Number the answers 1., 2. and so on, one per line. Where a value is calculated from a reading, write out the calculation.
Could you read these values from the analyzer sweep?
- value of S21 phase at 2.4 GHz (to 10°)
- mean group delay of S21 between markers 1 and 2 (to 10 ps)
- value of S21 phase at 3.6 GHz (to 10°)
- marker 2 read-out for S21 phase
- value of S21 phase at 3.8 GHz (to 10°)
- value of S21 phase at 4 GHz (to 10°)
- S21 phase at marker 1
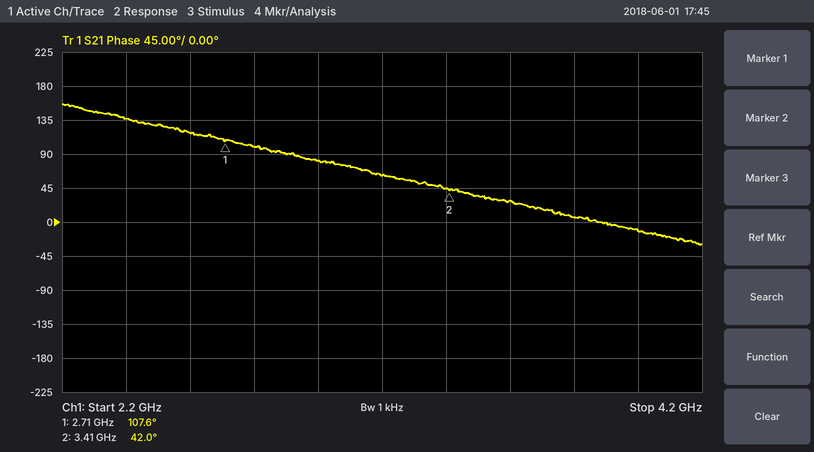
1. 140°
2. −(42° − (107.6°))/(360° × 700 MHz) ≈ 260 ps
3. 30°
4. 42.0°
5. 10°
6. -10°
7. 107.6°
